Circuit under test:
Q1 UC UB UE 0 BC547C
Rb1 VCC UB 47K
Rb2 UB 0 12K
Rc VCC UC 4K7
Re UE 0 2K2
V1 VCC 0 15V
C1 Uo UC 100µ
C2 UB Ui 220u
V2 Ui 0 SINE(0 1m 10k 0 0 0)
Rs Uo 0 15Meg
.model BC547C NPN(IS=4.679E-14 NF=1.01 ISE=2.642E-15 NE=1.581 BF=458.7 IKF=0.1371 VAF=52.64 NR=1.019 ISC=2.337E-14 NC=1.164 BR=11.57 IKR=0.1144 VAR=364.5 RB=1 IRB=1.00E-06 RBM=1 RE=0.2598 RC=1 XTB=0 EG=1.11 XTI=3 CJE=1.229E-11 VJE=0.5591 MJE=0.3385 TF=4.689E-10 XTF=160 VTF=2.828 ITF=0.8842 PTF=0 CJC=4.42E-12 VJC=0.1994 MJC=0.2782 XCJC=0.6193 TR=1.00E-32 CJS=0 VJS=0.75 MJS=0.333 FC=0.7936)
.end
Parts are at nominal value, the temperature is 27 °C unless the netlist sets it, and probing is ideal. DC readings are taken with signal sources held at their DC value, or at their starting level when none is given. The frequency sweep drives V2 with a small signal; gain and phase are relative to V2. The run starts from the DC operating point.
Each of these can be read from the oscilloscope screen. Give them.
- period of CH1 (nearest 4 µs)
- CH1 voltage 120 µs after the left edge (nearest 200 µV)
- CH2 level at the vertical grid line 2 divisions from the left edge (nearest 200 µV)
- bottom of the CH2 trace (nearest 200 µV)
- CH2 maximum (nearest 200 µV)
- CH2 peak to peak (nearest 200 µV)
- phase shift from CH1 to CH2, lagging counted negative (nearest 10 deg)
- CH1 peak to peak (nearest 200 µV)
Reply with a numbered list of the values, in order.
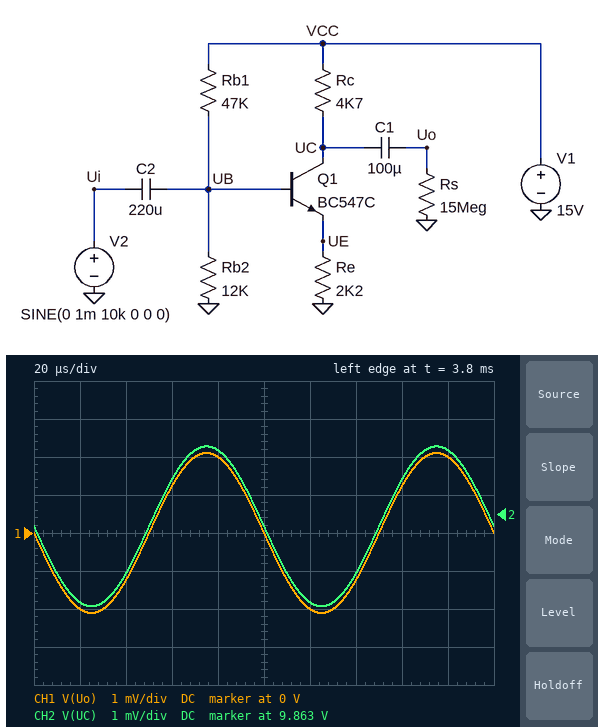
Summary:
1. 100 µs
2. -2.0 mV
3. 9.8614 V
4. 9.8606 V
5. 9.8648 V
6. 4.2 mV
7. 0 deg
8. 4.2 mV
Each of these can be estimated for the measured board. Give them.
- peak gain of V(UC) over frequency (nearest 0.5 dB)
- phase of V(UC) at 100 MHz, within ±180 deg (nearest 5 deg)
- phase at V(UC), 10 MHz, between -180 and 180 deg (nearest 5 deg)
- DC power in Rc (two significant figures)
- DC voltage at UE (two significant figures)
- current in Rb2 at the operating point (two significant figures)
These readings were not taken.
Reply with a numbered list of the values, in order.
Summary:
1. 6.5 dB
2. 25 deg
3. 135 deg
4. 5.6 mW
5. 2.4 V
6. 250 µA
